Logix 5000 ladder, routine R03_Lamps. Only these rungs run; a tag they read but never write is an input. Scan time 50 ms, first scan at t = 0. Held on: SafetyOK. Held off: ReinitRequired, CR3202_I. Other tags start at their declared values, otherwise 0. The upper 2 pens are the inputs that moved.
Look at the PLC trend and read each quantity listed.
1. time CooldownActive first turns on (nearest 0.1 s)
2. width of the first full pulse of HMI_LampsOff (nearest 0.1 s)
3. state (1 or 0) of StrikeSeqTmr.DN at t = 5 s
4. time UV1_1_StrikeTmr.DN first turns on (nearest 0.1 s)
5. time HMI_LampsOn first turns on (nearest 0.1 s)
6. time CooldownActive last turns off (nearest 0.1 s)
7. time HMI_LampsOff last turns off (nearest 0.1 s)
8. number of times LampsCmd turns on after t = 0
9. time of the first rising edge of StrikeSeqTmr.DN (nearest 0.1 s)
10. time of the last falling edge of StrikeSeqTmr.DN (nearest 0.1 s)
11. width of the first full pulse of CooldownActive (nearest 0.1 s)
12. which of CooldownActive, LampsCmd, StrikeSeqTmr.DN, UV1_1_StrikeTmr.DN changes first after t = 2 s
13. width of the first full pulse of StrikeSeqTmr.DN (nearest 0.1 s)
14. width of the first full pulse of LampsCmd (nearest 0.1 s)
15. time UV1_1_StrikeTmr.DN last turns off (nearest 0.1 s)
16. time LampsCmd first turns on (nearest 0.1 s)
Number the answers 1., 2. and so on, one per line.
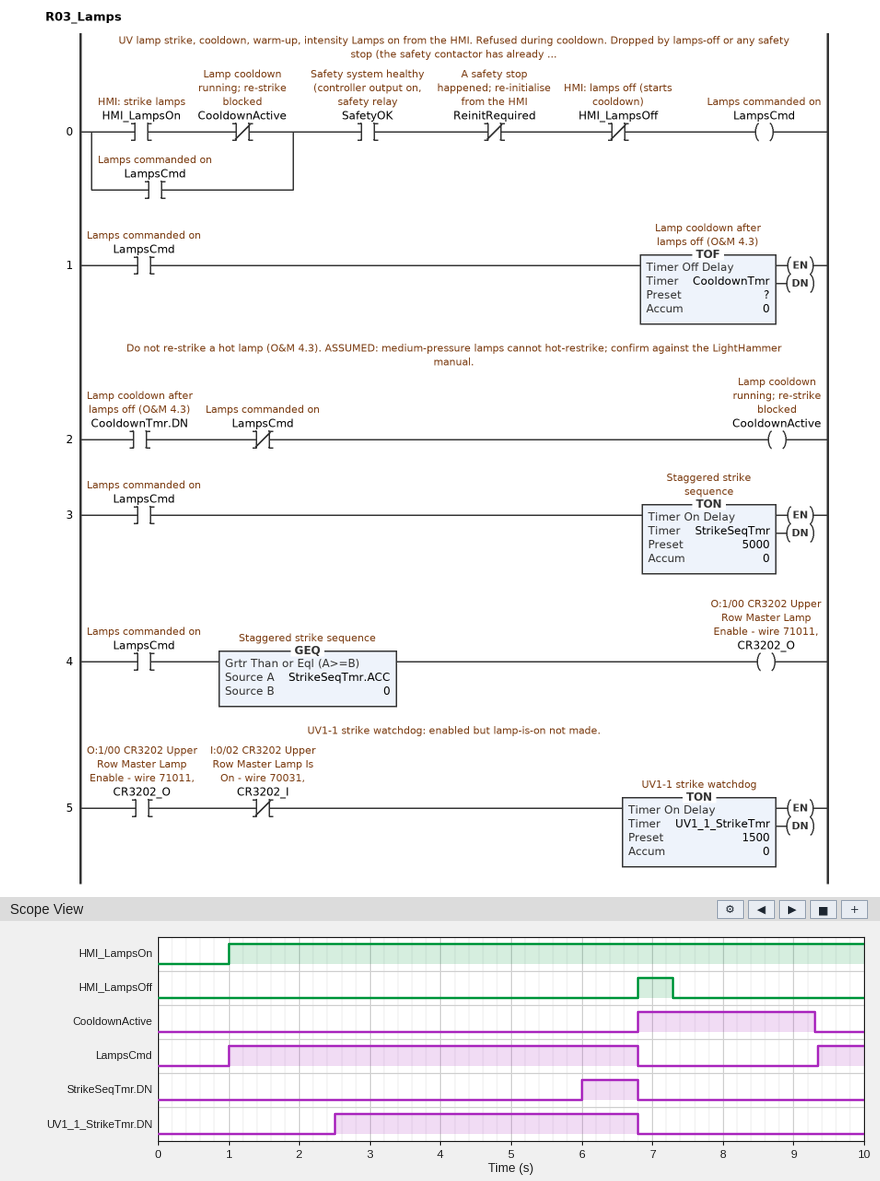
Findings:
1. 6.8 s
2. 0.5 s
3. 0
4. 2.5 s
5. 1.0 s
6. 9.3 s
7. 7.3 s
8. 2
9. 6.0 s
10. 6.8 s
11. 2.5 s
12. UV1_1_StrikeTmr.DN
13. 0.8 s
14. 5.8 s
15. 6.8 s
16. 1.0 s
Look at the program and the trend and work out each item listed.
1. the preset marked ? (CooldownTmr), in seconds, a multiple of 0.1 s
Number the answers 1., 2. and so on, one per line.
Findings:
1. 2.5 s
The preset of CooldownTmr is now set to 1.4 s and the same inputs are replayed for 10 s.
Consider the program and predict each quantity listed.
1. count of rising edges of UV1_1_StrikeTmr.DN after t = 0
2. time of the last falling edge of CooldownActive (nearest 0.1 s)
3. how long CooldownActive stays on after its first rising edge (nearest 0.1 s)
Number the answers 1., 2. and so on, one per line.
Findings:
1. 2
2. 8.2 s
3. 1.4 s
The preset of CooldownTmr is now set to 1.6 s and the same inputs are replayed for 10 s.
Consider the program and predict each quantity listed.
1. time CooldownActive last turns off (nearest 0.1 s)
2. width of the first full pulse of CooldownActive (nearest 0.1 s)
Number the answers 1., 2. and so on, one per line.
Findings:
1. 8.4 s
2. 1.6 s
